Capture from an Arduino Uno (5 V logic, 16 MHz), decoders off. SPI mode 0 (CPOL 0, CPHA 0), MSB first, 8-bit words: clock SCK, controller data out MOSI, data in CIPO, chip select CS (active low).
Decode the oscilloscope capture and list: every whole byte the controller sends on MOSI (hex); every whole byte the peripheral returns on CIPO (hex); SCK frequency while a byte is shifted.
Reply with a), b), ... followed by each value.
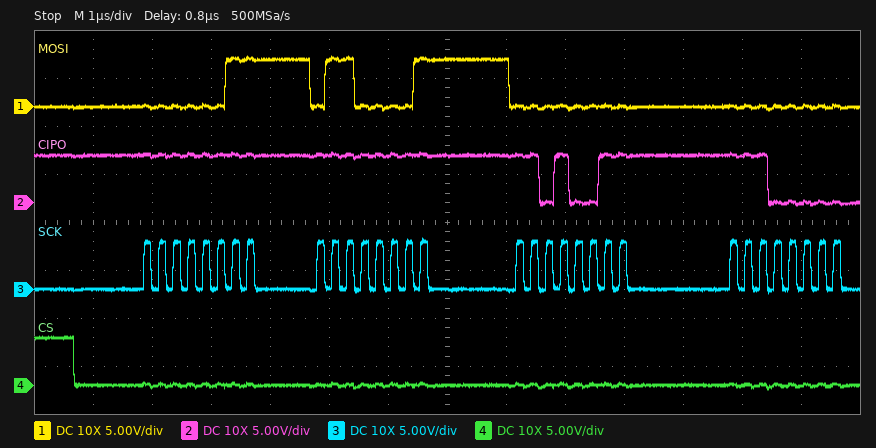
a) 03 61 00 00
b) FF FF D3 E0
c) 4 MHz
